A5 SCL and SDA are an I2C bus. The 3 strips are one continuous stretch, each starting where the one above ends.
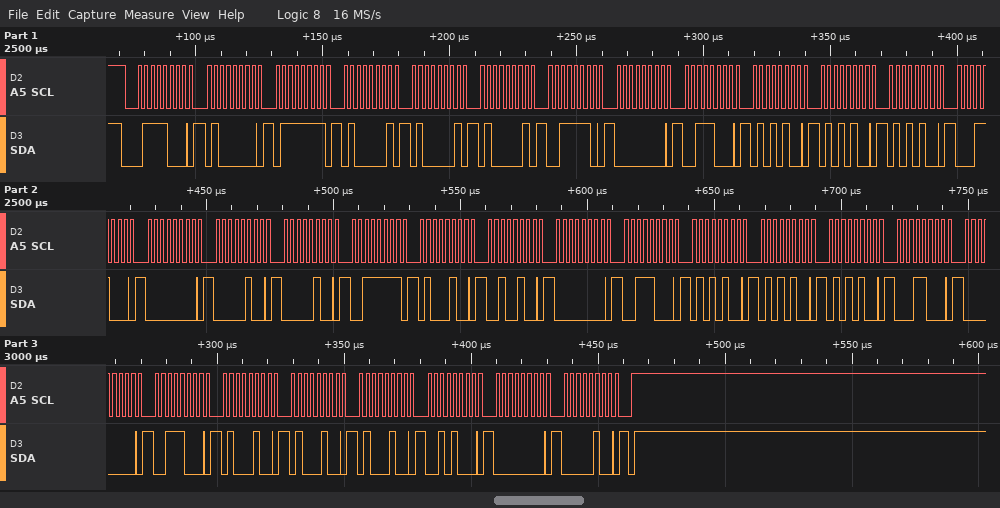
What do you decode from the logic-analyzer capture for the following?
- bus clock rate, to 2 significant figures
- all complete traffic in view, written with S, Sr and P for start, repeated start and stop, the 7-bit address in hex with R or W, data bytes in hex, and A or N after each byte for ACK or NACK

400 kHz
S 3CW A 40 A 7F A 41 A 41 A 41 A 3E A 00 A 38 A 54 A 54 A 54 A 18 A 00 A 04 A 04 A 3F A 44 A 24 A 00 A 38 A 54 A 54 A 54 A 18 A 00 A 38 A 44 A 44 A 44 A 28 A 00 A 04 A P
